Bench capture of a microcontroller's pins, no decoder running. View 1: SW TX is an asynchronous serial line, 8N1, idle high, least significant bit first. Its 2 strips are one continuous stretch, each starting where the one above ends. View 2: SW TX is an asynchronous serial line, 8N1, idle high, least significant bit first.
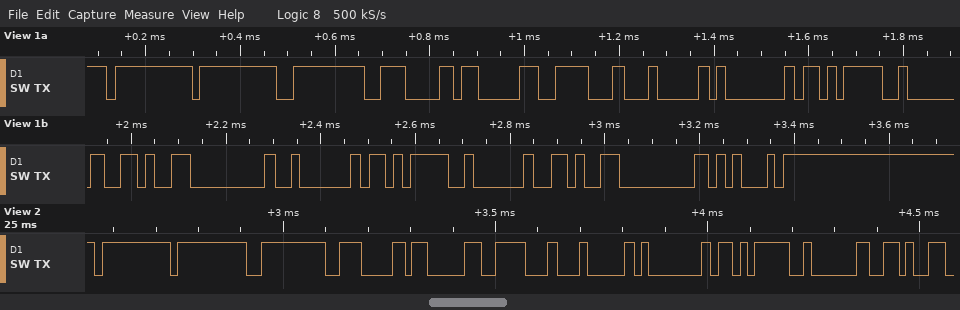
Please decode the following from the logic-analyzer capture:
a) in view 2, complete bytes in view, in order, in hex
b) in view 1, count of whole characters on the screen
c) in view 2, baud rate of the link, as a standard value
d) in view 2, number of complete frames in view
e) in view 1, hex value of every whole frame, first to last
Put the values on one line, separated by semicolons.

0xFF 0xFF 0xFE 0x0E 0x83 0x1E 0x04 0x01 0xEB 0x02 0x96; 18; 57600 baud; 11; FF FF FE 0E 83 1E 04 01 EB 02 96 00 02 EB 02 96 00 45
